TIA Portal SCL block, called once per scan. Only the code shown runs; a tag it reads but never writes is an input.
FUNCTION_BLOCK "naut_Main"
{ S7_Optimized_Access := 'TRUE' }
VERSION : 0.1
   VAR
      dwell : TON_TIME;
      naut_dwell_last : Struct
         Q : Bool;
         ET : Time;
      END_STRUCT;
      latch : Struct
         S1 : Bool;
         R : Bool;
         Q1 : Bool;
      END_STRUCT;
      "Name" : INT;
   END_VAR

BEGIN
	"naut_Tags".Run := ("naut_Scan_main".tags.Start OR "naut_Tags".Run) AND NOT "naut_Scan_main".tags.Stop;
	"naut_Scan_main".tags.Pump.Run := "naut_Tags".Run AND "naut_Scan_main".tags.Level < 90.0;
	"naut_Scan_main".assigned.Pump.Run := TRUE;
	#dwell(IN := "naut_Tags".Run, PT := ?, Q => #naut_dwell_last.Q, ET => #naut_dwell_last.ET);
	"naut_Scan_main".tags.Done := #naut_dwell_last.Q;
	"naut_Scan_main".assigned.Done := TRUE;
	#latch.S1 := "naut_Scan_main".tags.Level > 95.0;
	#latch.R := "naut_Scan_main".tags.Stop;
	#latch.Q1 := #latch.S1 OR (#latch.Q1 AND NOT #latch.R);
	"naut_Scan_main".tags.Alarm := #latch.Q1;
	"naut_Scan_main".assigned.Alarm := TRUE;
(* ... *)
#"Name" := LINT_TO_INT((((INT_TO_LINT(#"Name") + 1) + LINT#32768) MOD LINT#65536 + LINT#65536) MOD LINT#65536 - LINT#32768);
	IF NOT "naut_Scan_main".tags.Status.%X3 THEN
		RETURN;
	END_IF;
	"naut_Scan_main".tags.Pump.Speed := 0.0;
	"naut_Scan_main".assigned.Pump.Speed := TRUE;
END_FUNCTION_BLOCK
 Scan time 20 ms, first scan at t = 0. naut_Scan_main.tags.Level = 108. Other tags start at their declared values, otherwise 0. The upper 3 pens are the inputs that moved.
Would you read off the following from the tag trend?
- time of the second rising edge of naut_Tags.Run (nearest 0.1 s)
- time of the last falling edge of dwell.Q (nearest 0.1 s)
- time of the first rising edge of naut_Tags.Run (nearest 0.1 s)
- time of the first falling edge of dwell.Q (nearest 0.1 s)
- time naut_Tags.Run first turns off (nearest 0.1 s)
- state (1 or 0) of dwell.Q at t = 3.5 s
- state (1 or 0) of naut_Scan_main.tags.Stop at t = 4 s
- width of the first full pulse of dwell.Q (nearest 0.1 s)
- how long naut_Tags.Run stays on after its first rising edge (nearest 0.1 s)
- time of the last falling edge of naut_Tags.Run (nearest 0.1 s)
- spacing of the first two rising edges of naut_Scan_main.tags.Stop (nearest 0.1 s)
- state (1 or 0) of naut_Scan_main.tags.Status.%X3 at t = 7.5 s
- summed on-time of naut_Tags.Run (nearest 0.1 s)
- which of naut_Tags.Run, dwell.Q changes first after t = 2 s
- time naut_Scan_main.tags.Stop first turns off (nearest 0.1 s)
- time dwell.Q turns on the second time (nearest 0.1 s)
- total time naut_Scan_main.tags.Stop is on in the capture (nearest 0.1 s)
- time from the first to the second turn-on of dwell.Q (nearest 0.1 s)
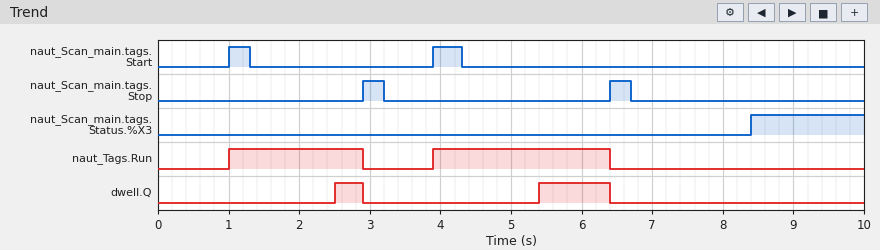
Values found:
3.9 s
6.4 s
1.0 s
2.9 s
2.9 s
0
0
0.4 s
1.9 s
6.4 s
3.5 s
0
4.4 s
dwell.Q
3.2 s
5.4 s
0.6 s
2.9 s
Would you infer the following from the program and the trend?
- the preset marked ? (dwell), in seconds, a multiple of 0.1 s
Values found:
1.5 s
